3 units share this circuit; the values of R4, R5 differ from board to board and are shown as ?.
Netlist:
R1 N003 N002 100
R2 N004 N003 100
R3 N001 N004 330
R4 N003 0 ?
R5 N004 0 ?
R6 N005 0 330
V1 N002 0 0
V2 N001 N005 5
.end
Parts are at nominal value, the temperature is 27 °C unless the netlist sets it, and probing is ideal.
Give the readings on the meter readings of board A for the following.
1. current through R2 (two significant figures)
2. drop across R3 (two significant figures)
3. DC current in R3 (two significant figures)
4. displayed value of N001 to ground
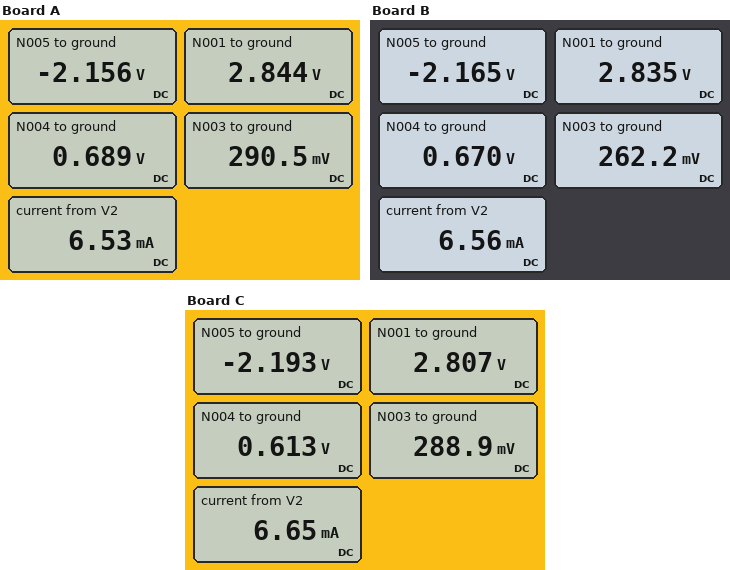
4.0 mA
2.2 V
6.5 mA
2.844 V
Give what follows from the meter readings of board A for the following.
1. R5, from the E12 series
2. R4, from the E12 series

270 Ω
270 Ω
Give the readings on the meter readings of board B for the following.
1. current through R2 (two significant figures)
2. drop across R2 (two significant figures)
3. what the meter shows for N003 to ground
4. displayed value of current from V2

4.1 mA
410 mV
262.2 mV
6.56 mA
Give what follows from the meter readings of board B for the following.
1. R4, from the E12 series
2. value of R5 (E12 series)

180 Ω
270 Ω
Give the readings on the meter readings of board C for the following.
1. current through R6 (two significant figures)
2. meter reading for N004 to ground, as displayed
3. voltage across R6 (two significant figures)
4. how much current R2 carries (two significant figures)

6.6 mA
0.613 V
2.2 V
3.2 mA
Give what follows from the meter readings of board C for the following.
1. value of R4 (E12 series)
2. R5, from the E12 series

820 Ω
180 Ω
